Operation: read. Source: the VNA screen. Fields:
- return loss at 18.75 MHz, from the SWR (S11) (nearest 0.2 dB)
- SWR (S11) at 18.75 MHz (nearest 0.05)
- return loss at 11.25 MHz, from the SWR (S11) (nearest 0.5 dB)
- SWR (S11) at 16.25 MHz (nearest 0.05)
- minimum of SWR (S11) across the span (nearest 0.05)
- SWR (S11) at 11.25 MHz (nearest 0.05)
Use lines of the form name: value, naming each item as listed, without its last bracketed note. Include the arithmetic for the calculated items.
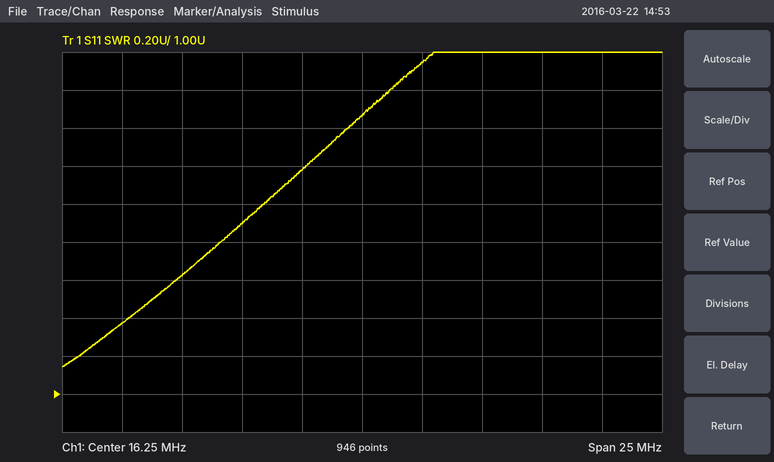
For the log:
return loss at 18.75 MHz, from the SWR (S11): −20 log10((2.75 − 1)/(2.75 + 1)) ≈ 6.6 dB
SWR (S11) at 18.75 MHz: 2.75
return loss at 11.25 MHz, from the SWR (S11): −20 log10((1.9 − 1)/(1.9 + 1)) ≈ 10.2 dB, so 10.0 dB to the nearest 0.5 dB
SWR (S11) at 16.25 MHz: 2.45
minimum of SWR (S11) across the span: 1.15
SWR (S11) at 11.25 MHz: 1.90
